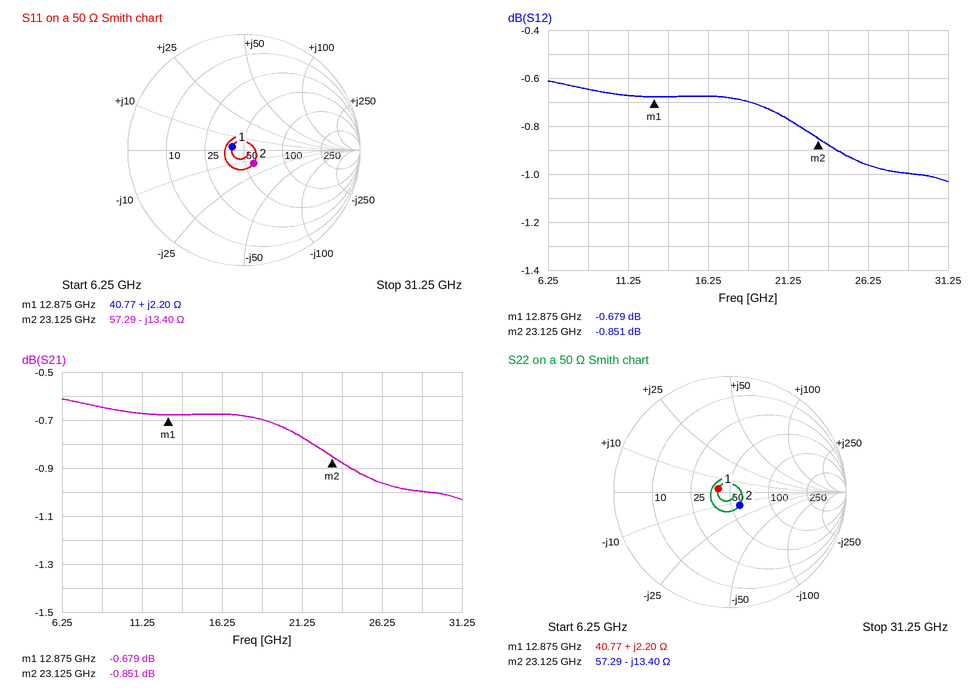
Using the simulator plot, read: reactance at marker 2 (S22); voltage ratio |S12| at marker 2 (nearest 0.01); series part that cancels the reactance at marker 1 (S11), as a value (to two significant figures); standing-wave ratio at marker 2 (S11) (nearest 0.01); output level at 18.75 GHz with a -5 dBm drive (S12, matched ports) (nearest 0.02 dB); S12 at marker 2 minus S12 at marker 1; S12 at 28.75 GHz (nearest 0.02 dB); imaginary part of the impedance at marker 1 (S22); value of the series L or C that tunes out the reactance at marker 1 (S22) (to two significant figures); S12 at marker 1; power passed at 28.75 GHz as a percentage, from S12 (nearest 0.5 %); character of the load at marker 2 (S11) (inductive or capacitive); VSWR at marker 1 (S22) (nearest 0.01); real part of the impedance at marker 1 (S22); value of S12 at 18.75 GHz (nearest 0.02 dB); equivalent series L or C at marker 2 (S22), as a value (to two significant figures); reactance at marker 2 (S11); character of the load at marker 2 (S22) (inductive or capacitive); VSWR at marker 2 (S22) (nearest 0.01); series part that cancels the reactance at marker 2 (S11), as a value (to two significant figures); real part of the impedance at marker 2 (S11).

-13.40 Ω
0.91
5.6 pF
1.33
-5.70 dBm
-0.172 dB
-1.00 dB
+2.20 Ω
5.6 pF
-0.679 dB
79.5 %
capacitive
1.23
40.77 Ω
-0.70 dB
510 fF
-13.40 Ω
capacitive
1.33
92 pH
57.29 Ω
